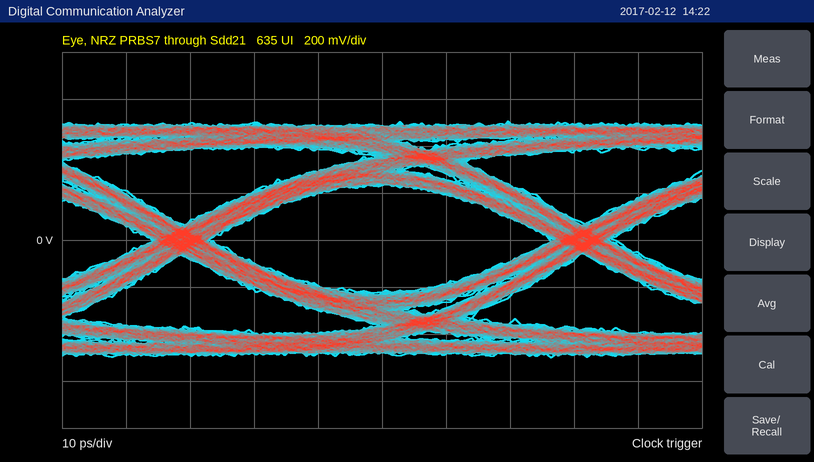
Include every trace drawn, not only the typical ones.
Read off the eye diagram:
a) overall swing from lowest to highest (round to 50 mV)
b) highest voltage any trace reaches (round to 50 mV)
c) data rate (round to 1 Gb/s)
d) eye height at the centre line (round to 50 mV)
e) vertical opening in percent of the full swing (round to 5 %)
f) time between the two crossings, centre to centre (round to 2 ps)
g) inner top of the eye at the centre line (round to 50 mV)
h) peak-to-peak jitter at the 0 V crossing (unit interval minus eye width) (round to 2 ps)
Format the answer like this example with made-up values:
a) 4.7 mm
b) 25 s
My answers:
a) 1.00 V
b) 500 mV
c) 16 Gb/s
d) 450 mV
e) 45 %
f) 62 ps
g) 250 mV
h) 10 ps
